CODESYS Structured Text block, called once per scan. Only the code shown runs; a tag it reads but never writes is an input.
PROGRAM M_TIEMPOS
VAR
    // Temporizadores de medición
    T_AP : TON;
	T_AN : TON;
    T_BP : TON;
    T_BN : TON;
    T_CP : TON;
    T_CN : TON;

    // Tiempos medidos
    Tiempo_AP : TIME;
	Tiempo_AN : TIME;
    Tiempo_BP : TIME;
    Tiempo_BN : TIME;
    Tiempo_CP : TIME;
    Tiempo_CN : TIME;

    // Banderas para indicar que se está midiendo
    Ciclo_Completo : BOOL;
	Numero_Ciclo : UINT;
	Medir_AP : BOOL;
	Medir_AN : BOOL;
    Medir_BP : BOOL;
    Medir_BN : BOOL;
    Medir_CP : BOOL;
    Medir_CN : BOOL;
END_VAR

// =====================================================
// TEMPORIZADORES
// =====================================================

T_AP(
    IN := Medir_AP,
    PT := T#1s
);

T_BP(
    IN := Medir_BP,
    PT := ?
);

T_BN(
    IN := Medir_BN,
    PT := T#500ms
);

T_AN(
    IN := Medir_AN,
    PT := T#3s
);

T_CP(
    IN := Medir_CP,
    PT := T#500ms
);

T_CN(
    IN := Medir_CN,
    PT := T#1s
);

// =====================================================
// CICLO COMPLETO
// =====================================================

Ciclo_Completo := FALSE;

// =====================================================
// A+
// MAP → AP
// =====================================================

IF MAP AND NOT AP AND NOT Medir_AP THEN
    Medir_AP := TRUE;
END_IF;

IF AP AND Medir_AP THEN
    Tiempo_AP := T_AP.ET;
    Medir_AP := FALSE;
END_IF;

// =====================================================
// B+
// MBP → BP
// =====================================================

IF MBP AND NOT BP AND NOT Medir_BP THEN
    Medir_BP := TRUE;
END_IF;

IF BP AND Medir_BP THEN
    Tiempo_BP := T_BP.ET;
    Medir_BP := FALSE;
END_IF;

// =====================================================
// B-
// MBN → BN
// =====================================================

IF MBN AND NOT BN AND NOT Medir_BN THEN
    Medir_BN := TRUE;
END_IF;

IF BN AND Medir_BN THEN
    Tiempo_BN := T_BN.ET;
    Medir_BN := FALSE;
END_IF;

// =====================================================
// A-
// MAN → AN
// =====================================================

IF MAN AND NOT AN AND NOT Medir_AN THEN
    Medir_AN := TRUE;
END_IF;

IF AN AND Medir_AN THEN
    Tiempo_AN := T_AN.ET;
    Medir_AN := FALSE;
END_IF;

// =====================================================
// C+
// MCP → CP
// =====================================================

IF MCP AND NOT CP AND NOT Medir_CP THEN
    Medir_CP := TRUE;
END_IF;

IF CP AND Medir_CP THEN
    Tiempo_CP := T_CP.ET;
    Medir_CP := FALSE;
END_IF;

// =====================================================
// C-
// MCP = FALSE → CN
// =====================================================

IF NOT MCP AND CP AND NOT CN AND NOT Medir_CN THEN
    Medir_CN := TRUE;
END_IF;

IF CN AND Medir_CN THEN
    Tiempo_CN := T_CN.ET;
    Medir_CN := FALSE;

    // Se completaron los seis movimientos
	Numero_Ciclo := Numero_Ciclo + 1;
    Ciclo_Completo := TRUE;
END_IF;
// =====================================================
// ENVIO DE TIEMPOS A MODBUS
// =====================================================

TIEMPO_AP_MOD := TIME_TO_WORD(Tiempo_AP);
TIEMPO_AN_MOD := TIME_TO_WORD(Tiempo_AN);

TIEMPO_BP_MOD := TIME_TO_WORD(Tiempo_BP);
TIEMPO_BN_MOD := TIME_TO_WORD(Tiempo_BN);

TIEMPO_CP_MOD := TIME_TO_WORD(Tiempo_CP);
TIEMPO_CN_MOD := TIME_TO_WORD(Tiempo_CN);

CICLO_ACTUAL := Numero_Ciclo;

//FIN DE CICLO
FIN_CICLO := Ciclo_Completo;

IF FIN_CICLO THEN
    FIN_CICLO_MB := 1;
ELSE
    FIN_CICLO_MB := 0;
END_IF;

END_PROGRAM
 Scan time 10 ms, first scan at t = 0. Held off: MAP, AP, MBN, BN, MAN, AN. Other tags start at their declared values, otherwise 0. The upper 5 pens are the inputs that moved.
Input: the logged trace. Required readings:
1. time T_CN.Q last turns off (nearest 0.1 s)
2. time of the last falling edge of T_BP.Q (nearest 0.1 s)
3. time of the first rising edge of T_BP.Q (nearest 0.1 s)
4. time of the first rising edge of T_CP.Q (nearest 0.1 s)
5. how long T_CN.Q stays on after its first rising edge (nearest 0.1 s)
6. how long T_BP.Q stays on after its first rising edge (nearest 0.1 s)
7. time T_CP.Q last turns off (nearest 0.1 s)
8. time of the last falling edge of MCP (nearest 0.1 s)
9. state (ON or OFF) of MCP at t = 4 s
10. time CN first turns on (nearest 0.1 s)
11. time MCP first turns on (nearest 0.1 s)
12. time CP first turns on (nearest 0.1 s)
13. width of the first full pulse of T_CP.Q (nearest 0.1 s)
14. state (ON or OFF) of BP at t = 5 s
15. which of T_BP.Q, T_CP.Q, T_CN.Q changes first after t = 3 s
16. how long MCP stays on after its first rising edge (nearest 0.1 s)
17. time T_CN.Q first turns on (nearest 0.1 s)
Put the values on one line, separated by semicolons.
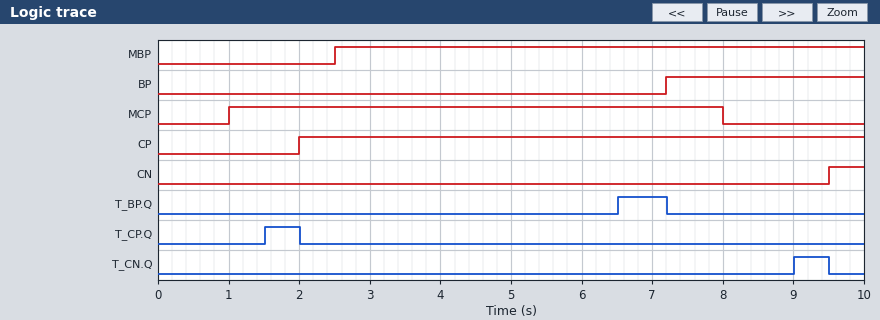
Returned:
9.5 s; 7.2 s; 6.5 s; 1.5 s; 0.5 s; 0.7 s; 2.0 s; 8.0 s; ON; 9.5 s; 1.0 s; 2.0 s; 0.5 s; OFF; T_BP.Q; 7.0 s; 9.0 s
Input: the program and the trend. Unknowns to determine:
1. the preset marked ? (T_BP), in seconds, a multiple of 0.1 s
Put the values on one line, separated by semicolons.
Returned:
4.0 s
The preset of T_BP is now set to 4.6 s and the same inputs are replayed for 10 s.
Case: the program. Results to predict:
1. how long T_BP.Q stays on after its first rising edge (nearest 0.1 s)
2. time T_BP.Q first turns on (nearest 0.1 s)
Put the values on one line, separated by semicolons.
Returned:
0.1 s; 7.1 s
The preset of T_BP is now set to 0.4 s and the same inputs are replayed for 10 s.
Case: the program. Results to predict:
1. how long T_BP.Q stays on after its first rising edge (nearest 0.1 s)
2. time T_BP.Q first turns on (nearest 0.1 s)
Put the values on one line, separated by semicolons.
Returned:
4.3 s; 2.9 s
